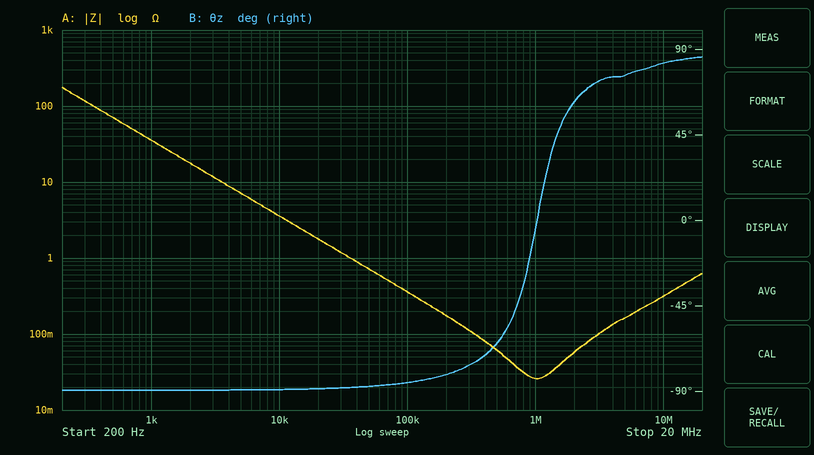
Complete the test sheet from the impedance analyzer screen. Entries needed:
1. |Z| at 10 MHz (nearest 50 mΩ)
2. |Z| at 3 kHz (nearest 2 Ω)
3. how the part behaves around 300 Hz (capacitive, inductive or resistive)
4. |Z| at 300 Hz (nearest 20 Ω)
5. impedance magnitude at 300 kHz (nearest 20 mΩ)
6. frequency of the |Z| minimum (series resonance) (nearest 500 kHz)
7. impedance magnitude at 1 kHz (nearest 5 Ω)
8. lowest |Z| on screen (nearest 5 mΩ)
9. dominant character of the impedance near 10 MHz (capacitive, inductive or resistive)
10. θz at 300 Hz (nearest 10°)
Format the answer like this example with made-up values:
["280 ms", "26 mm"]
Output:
["300 mΩ", "12 Ω", "capacitive", "120 Ω", "120 mΩ", "1.0 MHz", "35 Ω", "25 mΩ", "inductive", "-90°"]
